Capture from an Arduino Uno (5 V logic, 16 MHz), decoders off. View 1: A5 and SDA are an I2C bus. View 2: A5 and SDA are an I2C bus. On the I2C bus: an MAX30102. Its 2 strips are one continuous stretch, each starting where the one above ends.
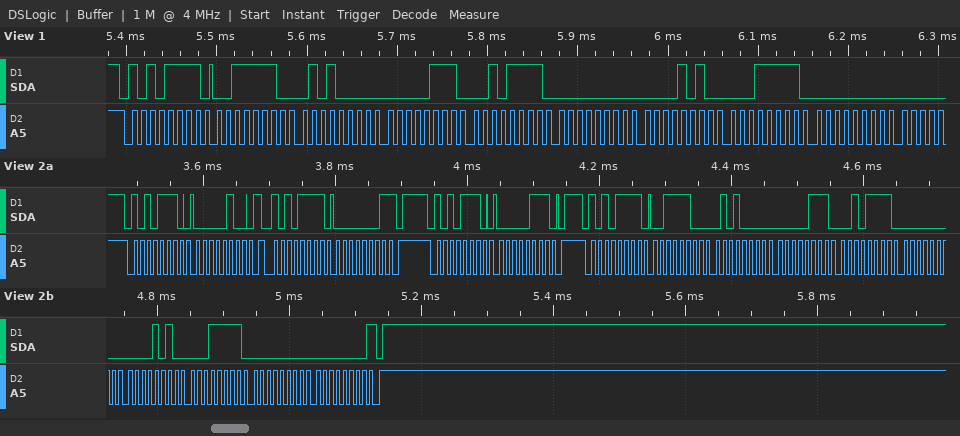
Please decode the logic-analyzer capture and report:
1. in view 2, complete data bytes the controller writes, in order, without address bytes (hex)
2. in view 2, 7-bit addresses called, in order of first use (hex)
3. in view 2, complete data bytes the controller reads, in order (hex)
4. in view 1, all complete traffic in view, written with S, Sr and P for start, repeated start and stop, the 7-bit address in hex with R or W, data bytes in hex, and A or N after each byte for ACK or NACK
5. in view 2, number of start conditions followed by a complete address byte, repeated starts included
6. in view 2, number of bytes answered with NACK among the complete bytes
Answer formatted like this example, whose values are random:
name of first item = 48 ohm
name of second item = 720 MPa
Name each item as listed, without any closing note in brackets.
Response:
in view 2, complete data bytes the controller writes, in order, without address bytes = 04 07
in view 2, 7-bit addresses called, in order of first use = 0x57
in view 2, complete data bytes the controller reads, in order = 01 3C 50 07 2F 00 0A 1F 00 00
in view 1, all complete traffic in view, written with S, Sr and P for start, repeated start and stop, the 7-bit address in hex with R or W, data bytes in hex, and A or N after each byte for ACK or NACK = S 57R A 3E A 50 A 07 A 2F A 00 A 0A A 1F A 00 A
in view 2, number of start conditions followed by a complete address byte, repeated starts included = 4
in view 2, number of bytes answered with NACK among the complete bytes = 2
